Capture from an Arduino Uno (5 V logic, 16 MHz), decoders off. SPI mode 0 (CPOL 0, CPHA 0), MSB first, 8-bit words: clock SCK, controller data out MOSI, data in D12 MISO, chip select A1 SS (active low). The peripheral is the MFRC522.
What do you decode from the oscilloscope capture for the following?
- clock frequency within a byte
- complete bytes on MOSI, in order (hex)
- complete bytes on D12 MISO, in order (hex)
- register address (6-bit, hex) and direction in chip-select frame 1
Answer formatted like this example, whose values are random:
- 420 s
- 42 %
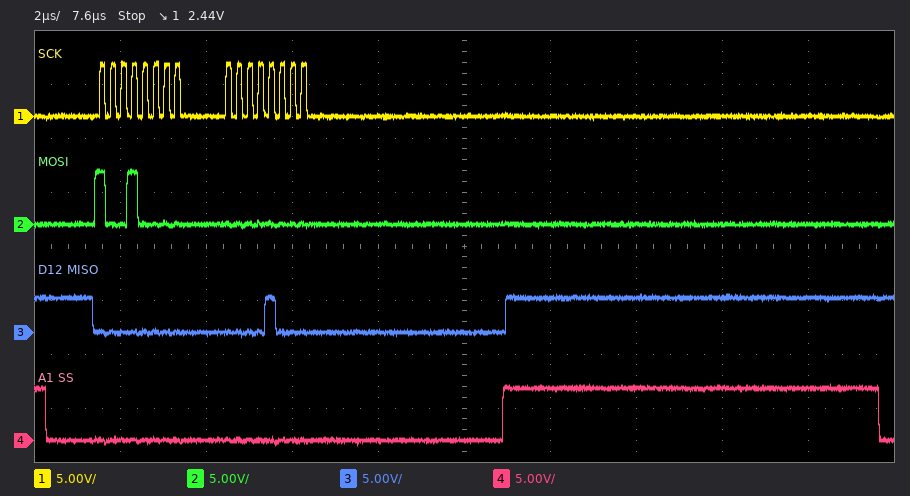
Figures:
- 4 MHz
- 90 00
- 00 08
- 0x08 read
